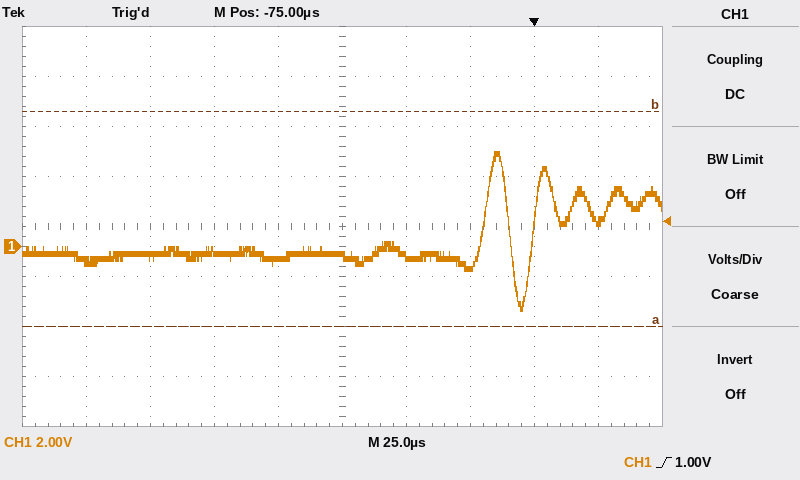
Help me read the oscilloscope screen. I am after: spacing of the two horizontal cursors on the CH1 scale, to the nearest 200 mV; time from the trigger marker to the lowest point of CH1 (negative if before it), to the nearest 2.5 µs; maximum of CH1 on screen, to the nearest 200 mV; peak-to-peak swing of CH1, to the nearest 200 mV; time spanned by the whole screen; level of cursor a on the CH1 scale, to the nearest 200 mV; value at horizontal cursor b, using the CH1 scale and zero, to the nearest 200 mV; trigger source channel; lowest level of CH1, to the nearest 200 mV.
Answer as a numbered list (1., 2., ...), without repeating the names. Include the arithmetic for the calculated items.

1. 8.6 V
2. -5.0 µs
3. 3.8 V
4. 3.8 V − (-2.6 V) = 6.4 V
5. 250 µs
6. -3.2 V
7. 5.4 V
8. CH1
9. -2.6 V
